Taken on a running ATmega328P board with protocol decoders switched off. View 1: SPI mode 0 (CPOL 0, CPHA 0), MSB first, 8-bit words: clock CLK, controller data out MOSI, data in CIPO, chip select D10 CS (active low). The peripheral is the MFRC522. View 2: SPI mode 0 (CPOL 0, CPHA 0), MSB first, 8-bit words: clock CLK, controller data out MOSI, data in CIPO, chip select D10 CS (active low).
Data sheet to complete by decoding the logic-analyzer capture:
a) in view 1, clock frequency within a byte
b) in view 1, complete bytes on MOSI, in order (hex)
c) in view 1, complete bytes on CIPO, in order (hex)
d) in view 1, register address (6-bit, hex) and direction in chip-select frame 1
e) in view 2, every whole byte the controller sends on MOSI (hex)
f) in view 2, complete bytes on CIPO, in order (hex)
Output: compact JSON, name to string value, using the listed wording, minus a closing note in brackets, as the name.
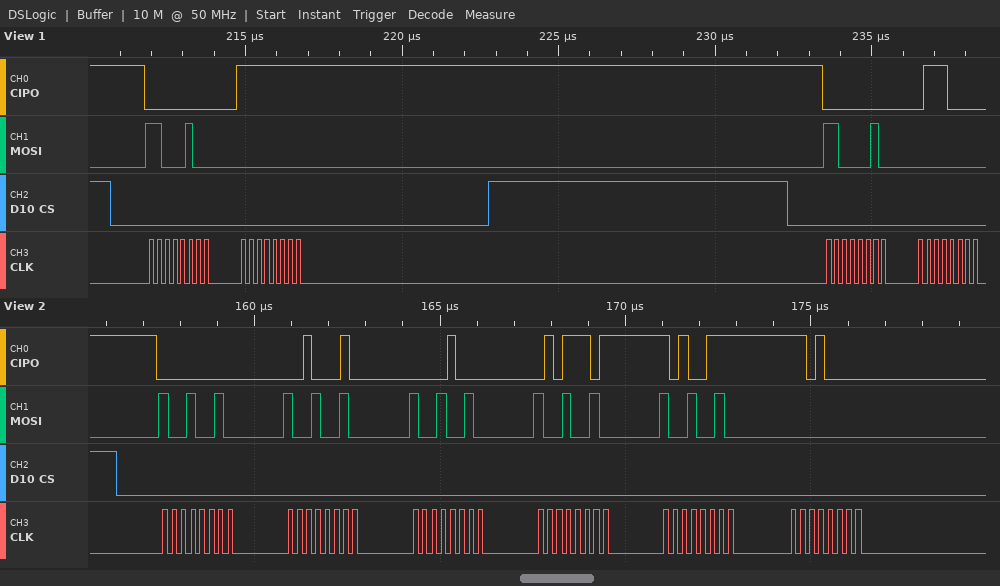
{"in view 1, clock frequency within a byte": "4 MHz", "in view 1, complete bytes on MOSI, in order": "C4 00 C2 00", "in view 1, complete bytes on CIPO, in order": "00 FF 00 70", "in view 1, register address (6-bit, hex) and direction in chip-select frame 1": "0x22 read", "in view 2, every whole byte the controller sends on MOSI": "92 92 92 92 92 00", "in view 2, complete bytes on CIPO, in order": "00 22 08 5D A7 D0"}
